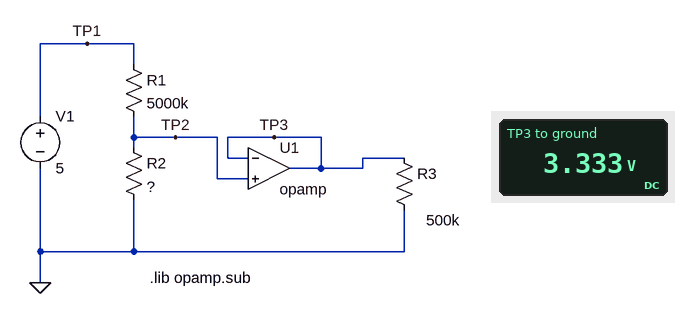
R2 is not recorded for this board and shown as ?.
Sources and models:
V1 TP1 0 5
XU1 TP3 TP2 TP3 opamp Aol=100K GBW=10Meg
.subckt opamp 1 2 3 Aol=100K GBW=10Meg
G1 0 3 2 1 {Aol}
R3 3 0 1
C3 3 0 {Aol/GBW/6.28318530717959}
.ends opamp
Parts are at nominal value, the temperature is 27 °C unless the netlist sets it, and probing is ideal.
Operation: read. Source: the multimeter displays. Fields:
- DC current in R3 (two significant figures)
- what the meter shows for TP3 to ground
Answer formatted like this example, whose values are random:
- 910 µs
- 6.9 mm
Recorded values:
- 6.7 µA
- 3.333 V
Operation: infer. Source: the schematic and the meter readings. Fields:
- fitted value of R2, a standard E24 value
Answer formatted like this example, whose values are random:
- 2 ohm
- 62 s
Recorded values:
- 10 MΩ
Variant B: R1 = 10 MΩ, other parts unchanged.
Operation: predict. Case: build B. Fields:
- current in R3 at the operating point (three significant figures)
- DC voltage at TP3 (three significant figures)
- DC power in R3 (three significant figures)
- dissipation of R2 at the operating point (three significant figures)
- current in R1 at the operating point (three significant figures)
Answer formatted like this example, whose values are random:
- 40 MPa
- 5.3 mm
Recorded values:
- 5.00 µA
- 2.50 V
- 12.5 µW
- 625 nW
- 250 nA
